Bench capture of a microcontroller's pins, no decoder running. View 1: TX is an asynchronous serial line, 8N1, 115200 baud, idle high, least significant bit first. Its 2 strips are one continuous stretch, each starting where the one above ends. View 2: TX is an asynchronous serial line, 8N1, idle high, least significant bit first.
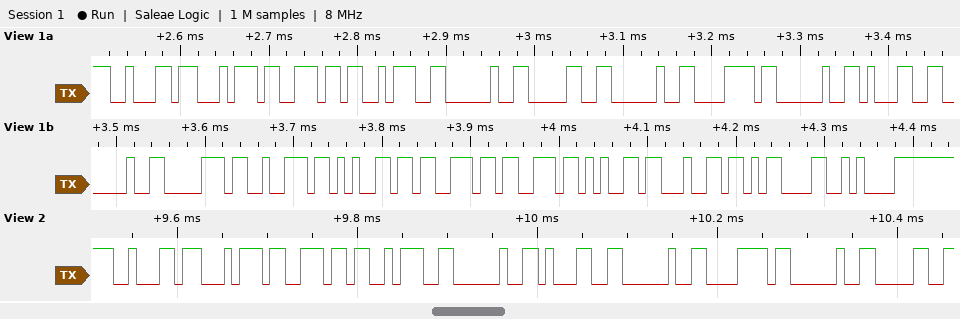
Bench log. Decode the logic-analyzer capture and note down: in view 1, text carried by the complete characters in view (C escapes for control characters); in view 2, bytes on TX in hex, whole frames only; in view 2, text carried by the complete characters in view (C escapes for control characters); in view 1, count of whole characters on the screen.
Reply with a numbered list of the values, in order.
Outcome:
1. "btn: 0 x 1 pressed\r\n"
2. 62 74 6E 3A 20 31 20 78 20 30
3. "btn: 1 x 0"
4. 20
